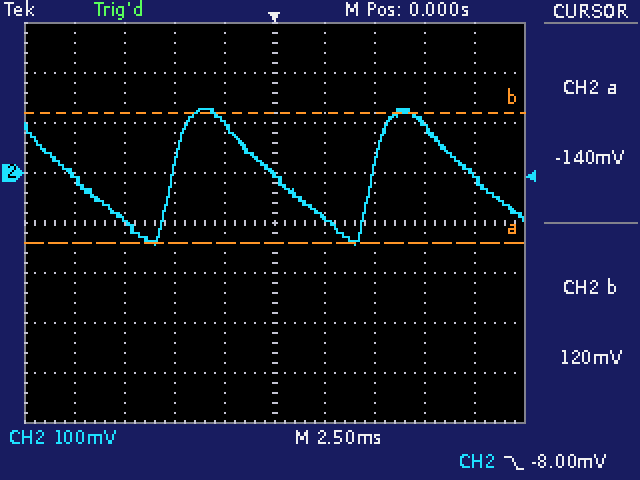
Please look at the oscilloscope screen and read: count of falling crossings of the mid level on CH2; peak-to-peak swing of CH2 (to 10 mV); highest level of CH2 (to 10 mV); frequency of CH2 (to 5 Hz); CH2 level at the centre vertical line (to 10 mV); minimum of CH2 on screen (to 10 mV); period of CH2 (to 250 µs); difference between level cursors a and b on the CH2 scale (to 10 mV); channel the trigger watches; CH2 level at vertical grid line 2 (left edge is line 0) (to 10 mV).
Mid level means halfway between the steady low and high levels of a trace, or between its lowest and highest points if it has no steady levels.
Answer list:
3
270 mV
130 mV
100 Hz
0 mV
-140 mV
10.00 ms
260 mV
CH2
-90 mV
